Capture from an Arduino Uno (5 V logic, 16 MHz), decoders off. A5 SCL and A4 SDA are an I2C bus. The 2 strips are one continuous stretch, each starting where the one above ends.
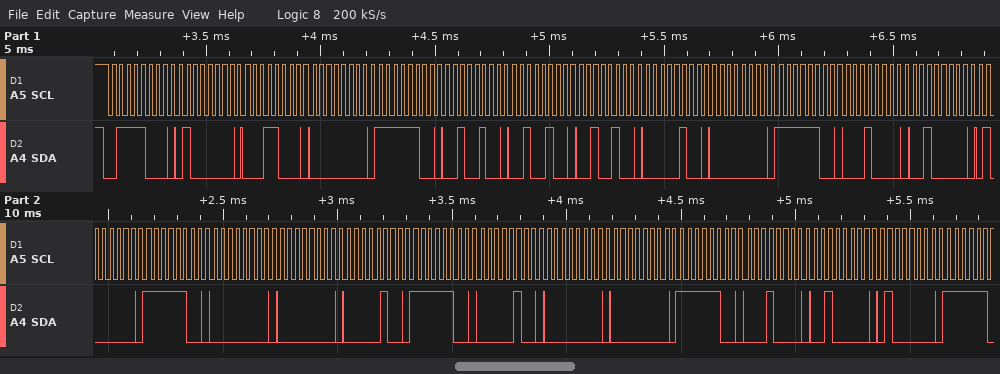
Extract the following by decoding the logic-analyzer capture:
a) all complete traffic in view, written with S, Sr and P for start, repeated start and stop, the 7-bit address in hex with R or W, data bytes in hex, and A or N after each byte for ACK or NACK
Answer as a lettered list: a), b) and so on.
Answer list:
a) S 3CW A 40 A 18 A 00 A FC A 24 A 24 A 24 A 04 A 00 A FC A 10 A 20 A 40 A FC A 00 A 00 A 04 A FC A 04 A 00 A 00 A FC A 10 A 20 A 40 A
